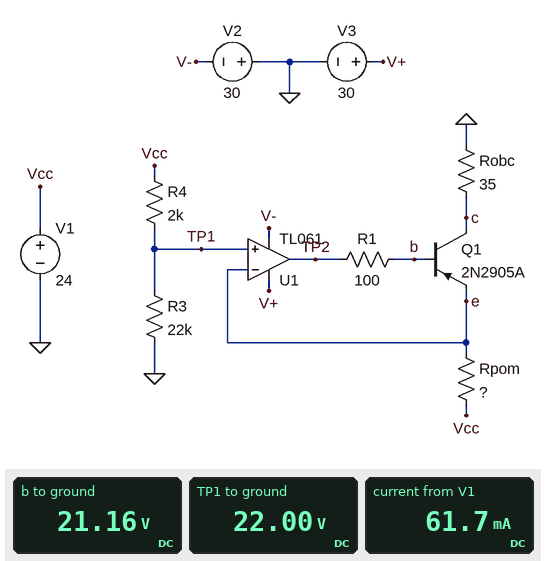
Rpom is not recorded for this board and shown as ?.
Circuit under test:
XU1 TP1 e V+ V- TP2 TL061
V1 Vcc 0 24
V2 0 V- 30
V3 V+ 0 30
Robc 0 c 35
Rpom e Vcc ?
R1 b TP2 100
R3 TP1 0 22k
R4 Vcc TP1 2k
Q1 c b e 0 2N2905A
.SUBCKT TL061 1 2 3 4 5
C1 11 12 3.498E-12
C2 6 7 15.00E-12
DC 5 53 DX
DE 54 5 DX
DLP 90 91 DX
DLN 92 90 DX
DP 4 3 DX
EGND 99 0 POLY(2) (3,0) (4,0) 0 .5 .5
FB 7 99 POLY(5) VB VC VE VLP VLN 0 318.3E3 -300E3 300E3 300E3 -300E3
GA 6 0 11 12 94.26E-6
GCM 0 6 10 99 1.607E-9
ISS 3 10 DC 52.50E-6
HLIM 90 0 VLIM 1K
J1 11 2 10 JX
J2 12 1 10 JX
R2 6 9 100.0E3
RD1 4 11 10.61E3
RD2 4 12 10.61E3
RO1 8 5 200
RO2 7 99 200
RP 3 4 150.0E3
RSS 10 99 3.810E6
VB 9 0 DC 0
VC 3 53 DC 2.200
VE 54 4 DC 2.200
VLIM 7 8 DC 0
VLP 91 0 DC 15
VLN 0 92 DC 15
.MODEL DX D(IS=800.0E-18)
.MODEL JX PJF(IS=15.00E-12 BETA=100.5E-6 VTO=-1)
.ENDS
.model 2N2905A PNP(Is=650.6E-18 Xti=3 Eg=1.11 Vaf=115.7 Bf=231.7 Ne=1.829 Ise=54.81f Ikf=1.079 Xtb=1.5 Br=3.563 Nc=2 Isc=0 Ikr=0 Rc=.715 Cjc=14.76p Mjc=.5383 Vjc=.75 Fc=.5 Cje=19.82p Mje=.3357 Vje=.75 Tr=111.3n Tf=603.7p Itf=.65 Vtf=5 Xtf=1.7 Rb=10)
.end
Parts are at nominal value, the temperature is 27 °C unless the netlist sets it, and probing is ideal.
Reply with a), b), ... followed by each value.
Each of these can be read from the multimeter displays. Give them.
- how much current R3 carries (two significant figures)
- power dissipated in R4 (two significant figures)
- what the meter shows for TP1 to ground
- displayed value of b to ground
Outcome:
a) 1.0 mA
b) 2.0 mW
c) 22.00 V
d) 21.16 V
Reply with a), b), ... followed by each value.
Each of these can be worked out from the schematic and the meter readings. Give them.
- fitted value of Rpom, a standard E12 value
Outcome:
a) 33 Ω
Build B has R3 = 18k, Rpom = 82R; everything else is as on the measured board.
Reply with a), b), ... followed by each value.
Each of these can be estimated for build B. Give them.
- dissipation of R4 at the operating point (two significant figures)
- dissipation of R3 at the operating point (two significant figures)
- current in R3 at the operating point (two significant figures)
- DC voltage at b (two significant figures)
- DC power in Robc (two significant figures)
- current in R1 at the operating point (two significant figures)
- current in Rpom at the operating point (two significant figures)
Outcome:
a) 2.9 mW
b) 26 mW
c) 1.2 mA
d) 21 V
e) 30 mW
f) 110 µA
g) 29 mA
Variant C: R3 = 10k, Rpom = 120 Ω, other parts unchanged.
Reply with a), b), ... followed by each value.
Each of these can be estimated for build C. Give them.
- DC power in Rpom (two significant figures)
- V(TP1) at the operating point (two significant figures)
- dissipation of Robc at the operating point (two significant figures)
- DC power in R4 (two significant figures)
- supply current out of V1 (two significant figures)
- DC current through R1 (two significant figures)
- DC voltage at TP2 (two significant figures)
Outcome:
a) 130 mW
b) 20 V
c) 39 mW
d) 8.0 mW
e) 35 mA
f) 130 µA
g) 19 V
